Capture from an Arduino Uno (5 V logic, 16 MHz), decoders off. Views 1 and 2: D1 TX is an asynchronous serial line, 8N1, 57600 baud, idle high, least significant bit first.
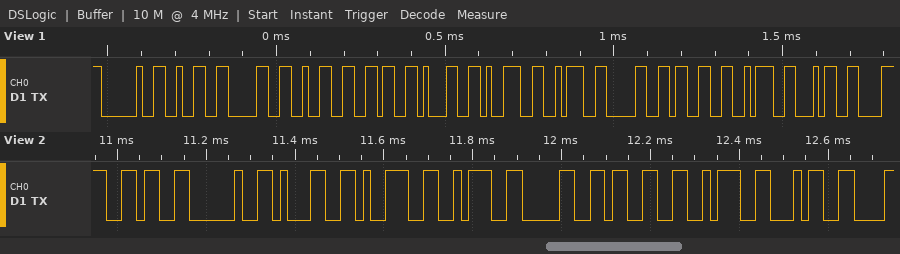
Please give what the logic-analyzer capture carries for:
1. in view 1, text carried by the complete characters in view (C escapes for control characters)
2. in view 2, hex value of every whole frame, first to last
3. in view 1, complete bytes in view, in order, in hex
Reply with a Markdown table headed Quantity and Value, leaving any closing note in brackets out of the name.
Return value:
| Quantity | Value |
|---|---|
| in view 1, text carried by the complete characters in view | " 202619:03:4" |
| in view 2, hex value of every whole frame, first to last | 36 20 31 39 3A 30 33 3A 34 |
| in view 1, complete bytes in view, in order, in hex | 20 32 30 32 36 31 39 3A 30 33 3A 34 |
